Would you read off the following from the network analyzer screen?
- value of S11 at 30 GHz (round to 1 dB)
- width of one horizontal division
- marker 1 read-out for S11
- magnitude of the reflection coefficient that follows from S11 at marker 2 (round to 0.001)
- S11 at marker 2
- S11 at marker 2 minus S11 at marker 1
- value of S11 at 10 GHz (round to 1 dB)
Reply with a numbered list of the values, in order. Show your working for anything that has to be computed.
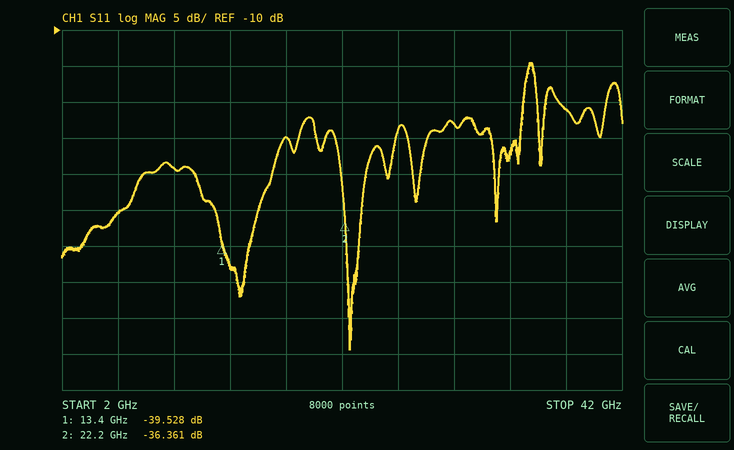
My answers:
1. -23 dB
2. 4 GHz
3. -39.528 dB
4. 10^(-36.361/20) ≈ 0.015
5. -36.361 dB
6. -36.361 − (-39.528) = 3.167 dB
7. -29 dB
